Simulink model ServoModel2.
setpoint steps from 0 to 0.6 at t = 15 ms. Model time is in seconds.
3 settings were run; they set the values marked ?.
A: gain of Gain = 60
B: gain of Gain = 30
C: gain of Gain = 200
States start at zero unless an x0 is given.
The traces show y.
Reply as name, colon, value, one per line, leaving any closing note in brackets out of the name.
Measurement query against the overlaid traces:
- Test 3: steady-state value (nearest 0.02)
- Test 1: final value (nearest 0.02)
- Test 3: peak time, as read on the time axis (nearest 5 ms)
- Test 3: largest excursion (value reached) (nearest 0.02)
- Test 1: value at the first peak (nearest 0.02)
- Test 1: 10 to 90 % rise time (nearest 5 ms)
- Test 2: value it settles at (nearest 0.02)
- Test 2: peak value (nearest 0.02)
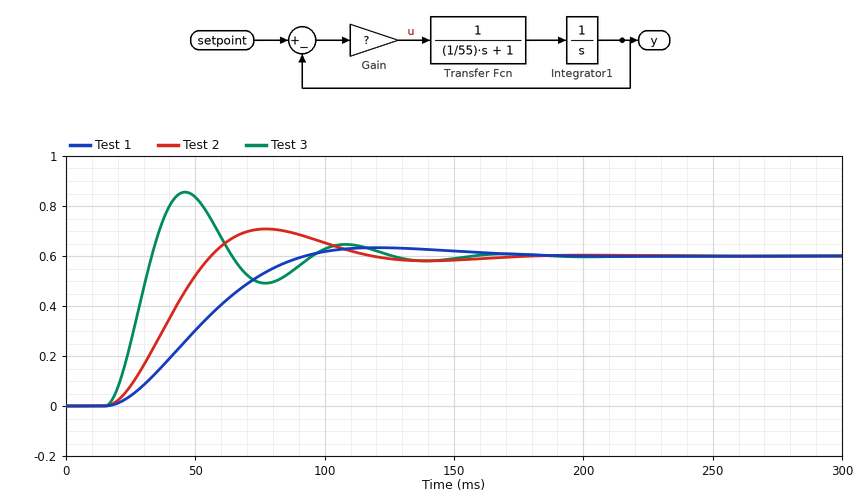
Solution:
Test 3: steady-state value: 0.60
Test 1: final value: 0.60
Test 3: peak time, as read on the time axis: 45 ms
Test 3: largest excursion (value reached): 0.86
Test 1: value at the first peak: 0.64
Test 1: 10 to 90 % rise time: 50 ms
Test 2: value it settles at: 0.60
Test 2: peak value: 0.70
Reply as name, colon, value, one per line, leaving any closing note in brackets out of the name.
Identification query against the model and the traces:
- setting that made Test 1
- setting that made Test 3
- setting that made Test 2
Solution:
setting that made Test 1: B
setting that made Test 3: C
setting that made Test 2: A
